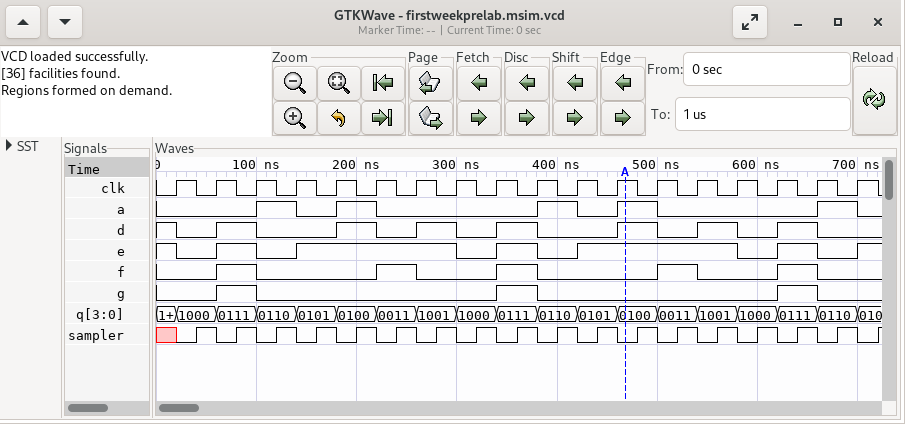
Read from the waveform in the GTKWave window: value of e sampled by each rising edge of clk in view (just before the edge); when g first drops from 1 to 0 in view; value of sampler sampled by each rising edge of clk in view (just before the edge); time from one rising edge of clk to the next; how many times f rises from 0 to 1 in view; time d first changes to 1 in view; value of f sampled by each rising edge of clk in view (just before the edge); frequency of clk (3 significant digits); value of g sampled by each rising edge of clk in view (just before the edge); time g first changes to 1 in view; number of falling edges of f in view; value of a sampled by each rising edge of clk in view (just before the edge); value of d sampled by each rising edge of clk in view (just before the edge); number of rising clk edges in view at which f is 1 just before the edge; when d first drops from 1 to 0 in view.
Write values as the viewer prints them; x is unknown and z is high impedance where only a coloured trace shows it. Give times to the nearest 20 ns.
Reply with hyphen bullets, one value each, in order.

- 1 0 1 0 1 1 1 1 0 1 0 1 1 1 1 0 1 0
- 100 ns
- x 1 1 1 1 1 1 1 1 1 1 1 1 1 1 1 1 1
- 40 ns
- 5
- 60 ns
- 0 0 1 0 0 0 1 0 0 1 0 0 0 1 0 0 1 0
- 25.0 MHz
- 0 0 1 0 0 0 0 0 0 1 0 0 0 0 0 0 1 0
- 60 ns
- 5
- 0 0 0 1 0 1 0 0 0 0 1 0 1 0 0 0 0 1
- 1 0 1 0 0 1 0 1 0 1 0 0 1 0 1 0 1 0
- 5
- 20 ns
